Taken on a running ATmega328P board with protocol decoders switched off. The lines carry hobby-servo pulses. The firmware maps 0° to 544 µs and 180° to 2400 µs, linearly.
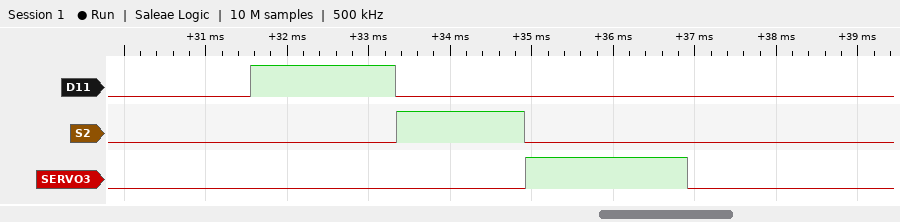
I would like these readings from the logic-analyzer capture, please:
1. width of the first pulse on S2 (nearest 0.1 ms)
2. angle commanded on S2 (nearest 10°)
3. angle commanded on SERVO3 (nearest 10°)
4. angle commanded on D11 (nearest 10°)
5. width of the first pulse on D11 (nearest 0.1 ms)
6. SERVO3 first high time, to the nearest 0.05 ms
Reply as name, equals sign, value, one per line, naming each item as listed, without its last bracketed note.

width of the first pulse on S2 = 1.6 ms
angle commanded on S2 = 100°
angle commanded on SERVO3 = 140°
angle commanded on D11 = 120°
width of the first pulse on D11 = 1.8 ms
SERVO3 first high time, to the nearest 0.05 ms = 2.00 ms
